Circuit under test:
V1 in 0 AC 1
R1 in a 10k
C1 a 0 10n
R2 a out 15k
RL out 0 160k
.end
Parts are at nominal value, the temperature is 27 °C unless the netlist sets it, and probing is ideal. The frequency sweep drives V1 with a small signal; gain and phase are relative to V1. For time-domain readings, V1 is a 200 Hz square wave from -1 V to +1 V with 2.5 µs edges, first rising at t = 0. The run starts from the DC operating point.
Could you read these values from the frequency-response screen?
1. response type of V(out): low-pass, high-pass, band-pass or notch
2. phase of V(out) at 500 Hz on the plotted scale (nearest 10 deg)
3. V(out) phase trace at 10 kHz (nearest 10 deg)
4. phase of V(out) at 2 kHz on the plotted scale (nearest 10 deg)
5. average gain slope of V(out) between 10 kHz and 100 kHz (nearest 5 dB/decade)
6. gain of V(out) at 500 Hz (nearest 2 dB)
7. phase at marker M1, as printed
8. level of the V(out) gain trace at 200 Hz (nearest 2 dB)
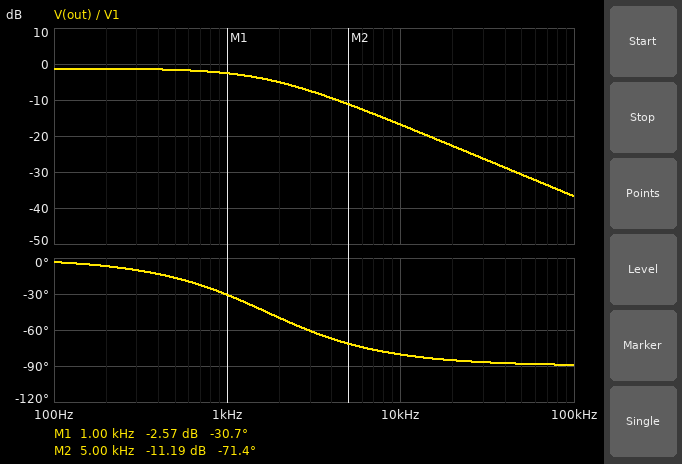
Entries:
low-pass
-20 deg
-80 deg
-50 deg
-20 dB/decade
-2 dB
-30.7 deg
-2 dB
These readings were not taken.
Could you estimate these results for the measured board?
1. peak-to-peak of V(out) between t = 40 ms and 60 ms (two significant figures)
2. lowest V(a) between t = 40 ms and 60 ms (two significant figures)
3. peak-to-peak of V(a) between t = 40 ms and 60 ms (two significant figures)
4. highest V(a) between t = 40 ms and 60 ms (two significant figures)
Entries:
1.7 V
-950 mV
1.9 V
950 mV
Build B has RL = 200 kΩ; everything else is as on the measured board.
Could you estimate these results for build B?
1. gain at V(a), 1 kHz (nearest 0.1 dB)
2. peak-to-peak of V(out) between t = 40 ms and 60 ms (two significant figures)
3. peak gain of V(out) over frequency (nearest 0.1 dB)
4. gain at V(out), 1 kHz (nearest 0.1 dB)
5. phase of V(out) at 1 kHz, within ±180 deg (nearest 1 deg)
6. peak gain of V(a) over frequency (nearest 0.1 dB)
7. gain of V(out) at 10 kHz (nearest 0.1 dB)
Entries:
-1.7 dB
1.8 V
-1.0 dB
-2.4 dB
-31 deg
-0.4 dB
-16.7 dB
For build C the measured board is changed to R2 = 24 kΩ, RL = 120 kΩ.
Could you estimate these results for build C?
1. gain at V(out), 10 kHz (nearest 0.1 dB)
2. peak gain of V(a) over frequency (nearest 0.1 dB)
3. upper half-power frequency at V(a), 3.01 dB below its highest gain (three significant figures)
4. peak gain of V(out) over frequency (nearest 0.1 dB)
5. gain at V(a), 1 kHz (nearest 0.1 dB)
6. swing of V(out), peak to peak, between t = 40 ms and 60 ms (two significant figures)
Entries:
-17.7 dB
-0.6 dB
1.70 kHz
-2.2 dB
-1.9 dB
1.6 V
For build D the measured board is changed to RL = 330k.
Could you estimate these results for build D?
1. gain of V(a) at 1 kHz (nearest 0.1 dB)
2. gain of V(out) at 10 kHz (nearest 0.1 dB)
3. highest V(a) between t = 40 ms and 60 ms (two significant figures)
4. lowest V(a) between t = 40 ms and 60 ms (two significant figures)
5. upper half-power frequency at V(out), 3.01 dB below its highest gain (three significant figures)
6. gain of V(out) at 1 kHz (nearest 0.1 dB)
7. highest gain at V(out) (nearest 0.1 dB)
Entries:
-1.6 dB
-16.5 dB
970 mV
-970 mV
1.64 kHz
-2.0 dB
-0.6 dB
